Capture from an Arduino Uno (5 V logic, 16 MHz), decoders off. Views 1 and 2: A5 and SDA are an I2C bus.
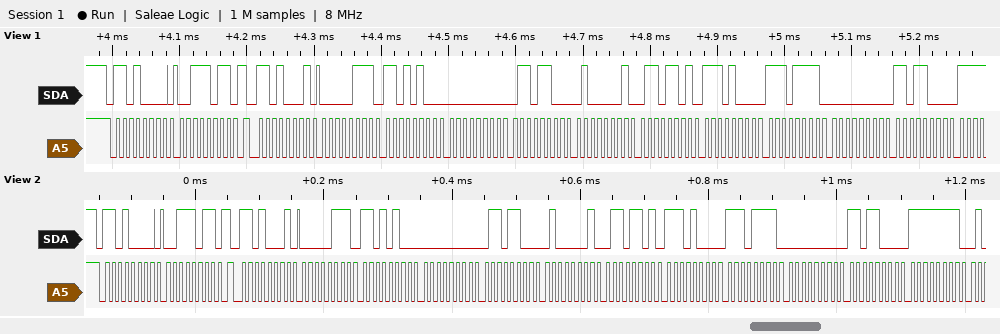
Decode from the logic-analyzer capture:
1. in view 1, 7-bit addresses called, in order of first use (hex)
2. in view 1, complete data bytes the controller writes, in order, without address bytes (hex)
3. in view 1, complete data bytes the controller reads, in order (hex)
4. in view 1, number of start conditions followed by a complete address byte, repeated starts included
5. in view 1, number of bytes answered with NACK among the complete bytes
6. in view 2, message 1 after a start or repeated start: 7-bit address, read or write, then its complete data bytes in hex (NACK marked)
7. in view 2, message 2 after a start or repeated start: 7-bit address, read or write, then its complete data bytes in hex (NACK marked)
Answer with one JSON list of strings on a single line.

["0x68", "3B", "07 D4 00 6C 41 6D E8 EF 00 D8", "2", "0", "0x68 write: 3B", "0x68 read: 07 D4 00 6C 41 6D E8 EF 00 D8 FF"]
